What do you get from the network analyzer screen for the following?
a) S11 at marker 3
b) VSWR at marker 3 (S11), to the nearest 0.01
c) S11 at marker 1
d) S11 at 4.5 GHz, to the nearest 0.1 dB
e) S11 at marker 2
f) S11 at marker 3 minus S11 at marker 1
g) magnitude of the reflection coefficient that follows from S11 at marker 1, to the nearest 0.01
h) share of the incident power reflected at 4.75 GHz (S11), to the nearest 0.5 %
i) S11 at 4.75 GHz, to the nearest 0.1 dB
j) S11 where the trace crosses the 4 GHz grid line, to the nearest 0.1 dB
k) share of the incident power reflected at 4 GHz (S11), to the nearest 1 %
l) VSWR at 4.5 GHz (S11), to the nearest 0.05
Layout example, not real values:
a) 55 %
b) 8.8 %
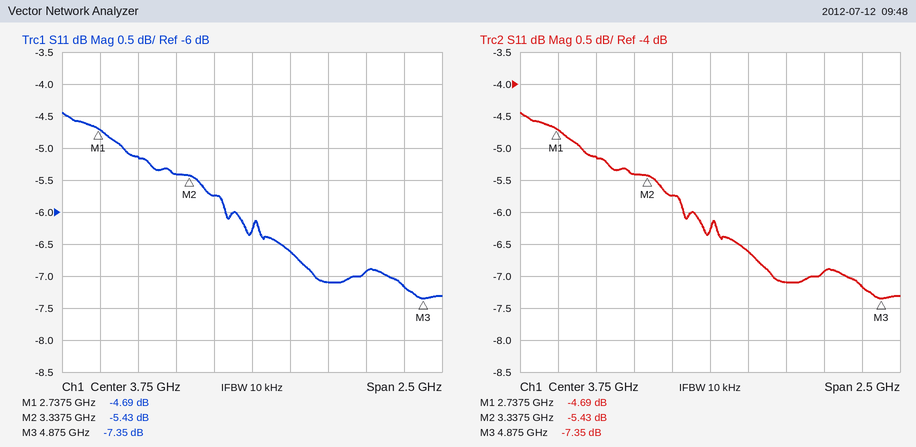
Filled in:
a) -7.35 dB
b) 2.50
c) -4.69 dB
d) -6.9 dB
e) -5.43 dB
f) -2.66 dB
g) 0.58
h) 19.0 %
i) -7.2 dB
j) -6.6 dB
k) 22 %
l) 2.65
